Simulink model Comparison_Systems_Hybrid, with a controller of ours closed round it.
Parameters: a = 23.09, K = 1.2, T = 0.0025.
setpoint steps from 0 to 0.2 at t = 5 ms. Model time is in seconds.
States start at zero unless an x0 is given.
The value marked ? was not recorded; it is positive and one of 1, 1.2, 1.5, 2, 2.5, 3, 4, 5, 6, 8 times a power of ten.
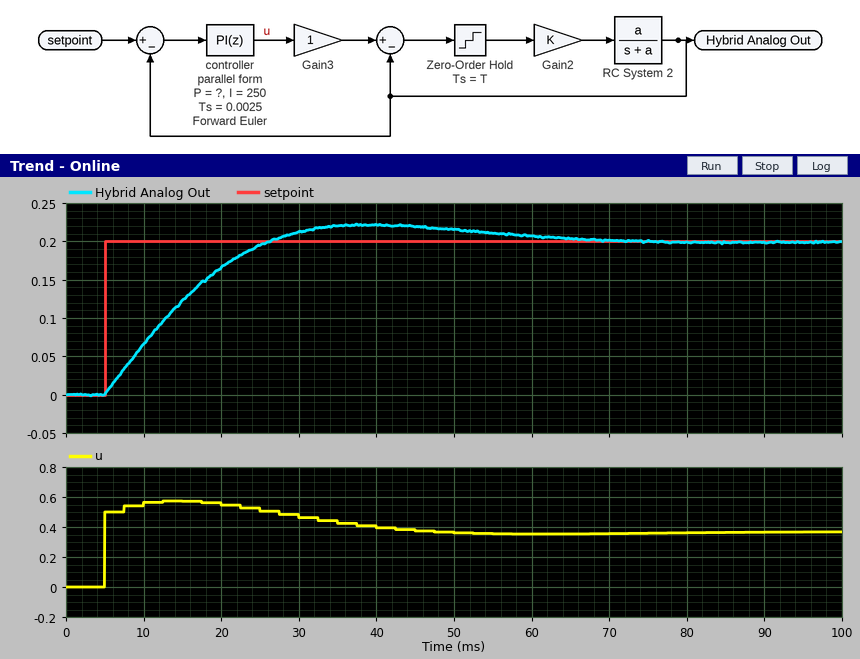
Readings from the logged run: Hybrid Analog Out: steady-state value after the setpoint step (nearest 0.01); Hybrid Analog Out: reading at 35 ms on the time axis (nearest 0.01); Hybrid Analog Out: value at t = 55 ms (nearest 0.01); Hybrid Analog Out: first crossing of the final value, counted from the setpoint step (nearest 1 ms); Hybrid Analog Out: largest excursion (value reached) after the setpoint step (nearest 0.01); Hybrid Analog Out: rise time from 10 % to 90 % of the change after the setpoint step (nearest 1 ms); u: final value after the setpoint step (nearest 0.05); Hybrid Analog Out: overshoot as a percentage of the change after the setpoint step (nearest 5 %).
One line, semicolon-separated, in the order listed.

0.20; 0.22; 0.21; 21 ms; 0.22; 16 ms; 0.35; 10 %
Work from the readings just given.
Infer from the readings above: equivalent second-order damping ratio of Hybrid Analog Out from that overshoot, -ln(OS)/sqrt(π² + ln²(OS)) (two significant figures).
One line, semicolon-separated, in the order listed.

0.59
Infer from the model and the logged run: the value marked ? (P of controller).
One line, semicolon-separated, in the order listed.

2.5
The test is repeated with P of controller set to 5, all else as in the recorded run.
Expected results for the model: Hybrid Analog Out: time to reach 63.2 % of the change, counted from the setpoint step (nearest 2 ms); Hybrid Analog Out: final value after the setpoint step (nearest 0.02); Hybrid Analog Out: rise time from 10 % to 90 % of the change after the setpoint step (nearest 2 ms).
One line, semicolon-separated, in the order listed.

6 ms; 0.20; 14 ms
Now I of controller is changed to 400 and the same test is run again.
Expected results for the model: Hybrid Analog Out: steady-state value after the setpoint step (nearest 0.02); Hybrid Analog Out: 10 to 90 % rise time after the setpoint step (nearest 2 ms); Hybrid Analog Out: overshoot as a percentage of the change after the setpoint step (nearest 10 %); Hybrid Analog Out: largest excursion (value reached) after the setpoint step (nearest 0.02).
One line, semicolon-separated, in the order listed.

0.20; 12 ms; 20 %; 0.24
